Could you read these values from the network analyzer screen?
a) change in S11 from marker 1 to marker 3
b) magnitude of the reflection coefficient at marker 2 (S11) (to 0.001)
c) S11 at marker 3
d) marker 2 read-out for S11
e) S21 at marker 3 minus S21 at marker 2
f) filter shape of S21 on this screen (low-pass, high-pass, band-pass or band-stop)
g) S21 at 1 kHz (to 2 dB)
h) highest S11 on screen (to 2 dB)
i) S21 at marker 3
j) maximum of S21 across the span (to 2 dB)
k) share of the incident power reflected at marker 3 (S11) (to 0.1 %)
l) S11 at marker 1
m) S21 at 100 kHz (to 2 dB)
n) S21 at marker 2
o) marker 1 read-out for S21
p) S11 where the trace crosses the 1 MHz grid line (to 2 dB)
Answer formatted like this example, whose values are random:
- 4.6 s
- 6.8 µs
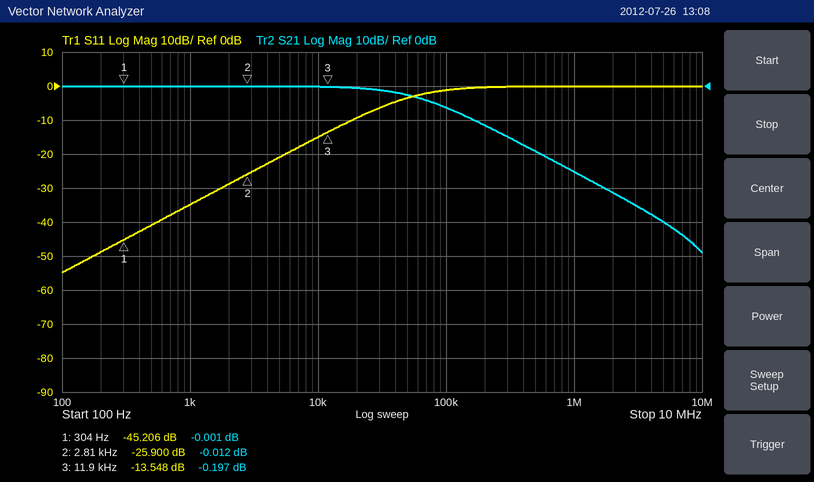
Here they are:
- 31.658 dB
- 0.051
- -13.548 dB
- -25.900 dB
- -0.185 dB
- low-pass
- 0 dB
- 0 dB
- -0.197 dB
- 0 dB
- 4.4 %
- -45.206 dB
- -6 dB
- -0.012 dB
- -0.001 dB
- 0 dB
